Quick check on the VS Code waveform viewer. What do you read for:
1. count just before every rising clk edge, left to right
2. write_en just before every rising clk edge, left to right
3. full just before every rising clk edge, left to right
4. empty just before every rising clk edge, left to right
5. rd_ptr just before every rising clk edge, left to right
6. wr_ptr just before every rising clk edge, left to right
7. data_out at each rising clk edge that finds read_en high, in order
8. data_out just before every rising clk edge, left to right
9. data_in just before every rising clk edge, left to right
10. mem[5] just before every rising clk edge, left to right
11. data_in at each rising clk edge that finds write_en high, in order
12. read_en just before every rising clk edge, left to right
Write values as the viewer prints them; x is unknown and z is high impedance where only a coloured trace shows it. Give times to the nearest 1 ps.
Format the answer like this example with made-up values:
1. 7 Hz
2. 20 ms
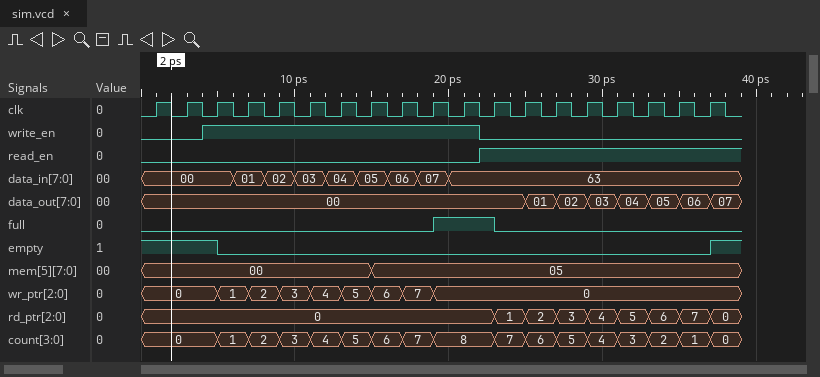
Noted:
1. 0, 0, 0, 1, 2, 3, 4, 5, 6, 7, 8, 8, 7, 6, 5, 4, 3, 2, 1
2. 0 0 1 1 1 1 1 1 1 1 1 0 0 0 0 0 0 0 0
3. 0 0 0 0 0 0 0 0 0 0 1 1 0 0 0 0 0 0 0
4. 1 1 1 0 0 0 0 0 0 0 0 0 0 0 0 0 0 0 0
5. 0, 0, 0, 0, 0, 0, 0, 0, 0, 0, 0, 0, 1, 2, 3, 4, 5, 6, 7
6. 0, 0, 0, 1, 2, 3, 4, 5, 6, 7, 0, 0, 0, 0, 0, 0, 0, 0, 0
7. 00, 00, 01, 02, 03, 04, 05, 06
8. 00, 00, 00, 00, 00, 00, 00, 00, 00, 00, 00, 00, 00, 01, 02, 03, 04, 05, 06
9. 00, 00, 00, 01, 02, 03, 04, 05, 06, 07, 63, 63, 63, 63, 63, 63, 63, 63, 63
10. 00, 00, 00, 00, 00, 00, 00, 00, 05, 05, 05, 05, 05, 05, 05, 05, 05, 05, 05
11. 00, 01, 02, 03, 04, 05, 06, 07, 63
12. 0 0 0 0 0 0 0 0 0 0 0 1 1 1 1 1 1 1 1
